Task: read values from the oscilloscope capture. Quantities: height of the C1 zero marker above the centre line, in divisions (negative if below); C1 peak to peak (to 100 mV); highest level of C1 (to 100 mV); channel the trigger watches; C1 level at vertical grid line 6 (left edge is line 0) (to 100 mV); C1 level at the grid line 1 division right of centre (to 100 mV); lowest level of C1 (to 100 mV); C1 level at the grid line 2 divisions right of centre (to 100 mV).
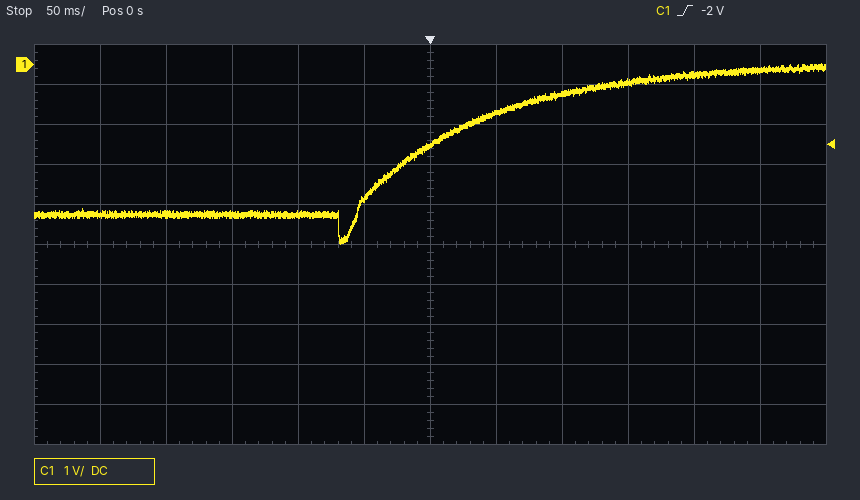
+4.5 div
4.5 V
0.0 V
C1
-2.0 V
-1.2 V
-4.5 V
-700 mV
